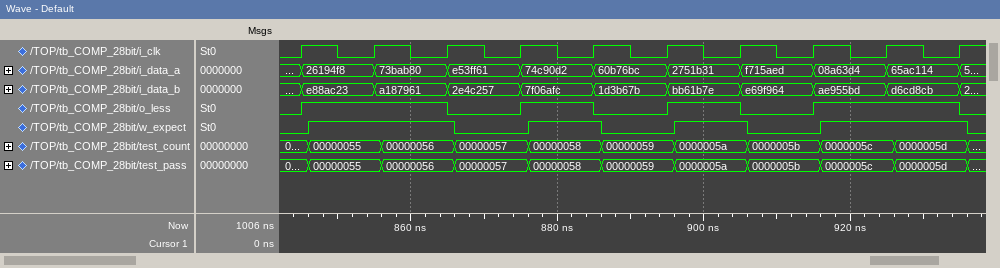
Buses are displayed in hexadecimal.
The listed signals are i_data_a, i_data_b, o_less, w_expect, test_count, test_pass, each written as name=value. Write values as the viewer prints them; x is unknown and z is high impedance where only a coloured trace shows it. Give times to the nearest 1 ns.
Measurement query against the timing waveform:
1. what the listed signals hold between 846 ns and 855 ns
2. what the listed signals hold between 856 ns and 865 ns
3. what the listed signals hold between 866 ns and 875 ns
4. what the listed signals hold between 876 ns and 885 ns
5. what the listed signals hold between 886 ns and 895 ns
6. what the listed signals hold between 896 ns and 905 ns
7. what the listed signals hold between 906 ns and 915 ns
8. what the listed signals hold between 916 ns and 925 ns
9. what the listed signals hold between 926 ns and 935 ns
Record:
i_data_a=26194f8, i_data_b=e88ac23, o_less=1, w_expect=1, test_count=00000055, test_pass=00000055
i_data_a=73bab80, i_data_b=a187961, o_less=1, w_expect=1, test_count=00000056, test_pass=00000056
i_data_a=e53ff61, i_data_b=2e4c257, o_less=0, w_expect=0, test_count=00000057, test_pass=00000057
i_data_a=74c90d2, i_data_b=7f06afc, o_less=1, w_expect=1, test_count=00000058, test_pass=00000058
i_data_a=60b76bc, i_data_b=1d3b67b, o_less=0, w_expect=0, test_count=00000059, test_pass=00000059
i_data_a=2751b31, i_data_b=bb61b7e, o_less=1, w_expect=1, test_count=0000005a, test_pass=0000005a
i_data_a=f715aed, i_data_b=e69f964, o_less=0, w_expect=0, test_count=0000005b, test_pass=0000005b
i_data_a=08a63d4, i_data_b=ae955bd, o_less=1, w_expect=1, test_count=0000005c, test_pass=0000005c
i_data_a=65ac114, i_data_b=d6cd8cb, o_less=1, w_expect=1, test_count=0000005d, test_pass=0000005d
